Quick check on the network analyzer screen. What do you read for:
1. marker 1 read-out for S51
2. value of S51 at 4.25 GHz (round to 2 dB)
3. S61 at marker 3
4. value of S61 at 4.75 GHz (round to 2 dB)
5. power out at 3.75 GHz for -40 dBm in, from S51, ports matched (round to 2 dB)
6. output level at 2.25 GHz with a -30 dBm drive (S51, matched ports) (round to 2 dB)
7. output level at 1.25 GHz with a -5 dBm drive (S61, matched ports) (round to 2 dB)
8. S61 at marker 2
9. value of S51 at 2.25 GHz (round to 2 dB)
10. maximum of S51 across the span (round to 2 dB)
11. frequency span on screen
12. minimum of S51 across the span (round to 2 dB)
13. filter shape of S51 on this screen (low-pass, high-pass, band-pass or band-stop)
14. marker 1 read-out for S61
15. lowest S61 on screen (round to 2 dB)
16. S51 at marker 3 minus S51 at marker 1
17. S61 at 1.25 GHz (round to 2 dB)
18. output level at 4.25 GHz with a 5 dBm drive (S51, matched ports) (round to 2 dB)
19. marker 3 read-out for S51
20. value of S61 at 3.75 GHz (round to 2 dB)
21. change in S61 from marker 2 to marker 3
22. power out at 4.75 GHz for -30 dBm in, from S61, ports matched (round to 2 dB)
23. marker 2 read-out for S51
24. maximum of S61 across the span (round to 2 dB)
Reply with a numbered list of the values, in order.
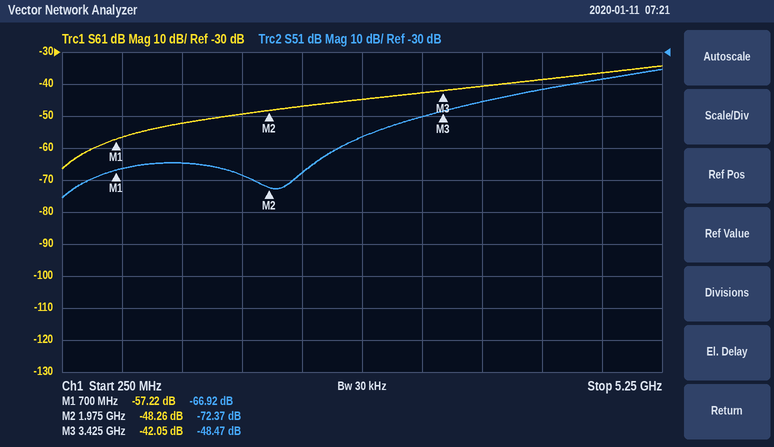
1. -66.92 dB
2. -42 dB
3. -42.05 dB
4. -36 dB
5. -86 dBm
6. -98 dBm
7. -58 dBm
8. -48.26 dB
9. -68 dB
10. -36 dB
11. 5 GHz
12. -76 dB
13. high-pass
14. -57.22 dB
15. -66 dB
16. 18.45 dB
17. -52 dB
18. -36 dBm
19. -48.47 dB
20. -40 dB
21. 6.21 dB
22. -66 dBm
23. -72.37 dB
24. -34 dB
